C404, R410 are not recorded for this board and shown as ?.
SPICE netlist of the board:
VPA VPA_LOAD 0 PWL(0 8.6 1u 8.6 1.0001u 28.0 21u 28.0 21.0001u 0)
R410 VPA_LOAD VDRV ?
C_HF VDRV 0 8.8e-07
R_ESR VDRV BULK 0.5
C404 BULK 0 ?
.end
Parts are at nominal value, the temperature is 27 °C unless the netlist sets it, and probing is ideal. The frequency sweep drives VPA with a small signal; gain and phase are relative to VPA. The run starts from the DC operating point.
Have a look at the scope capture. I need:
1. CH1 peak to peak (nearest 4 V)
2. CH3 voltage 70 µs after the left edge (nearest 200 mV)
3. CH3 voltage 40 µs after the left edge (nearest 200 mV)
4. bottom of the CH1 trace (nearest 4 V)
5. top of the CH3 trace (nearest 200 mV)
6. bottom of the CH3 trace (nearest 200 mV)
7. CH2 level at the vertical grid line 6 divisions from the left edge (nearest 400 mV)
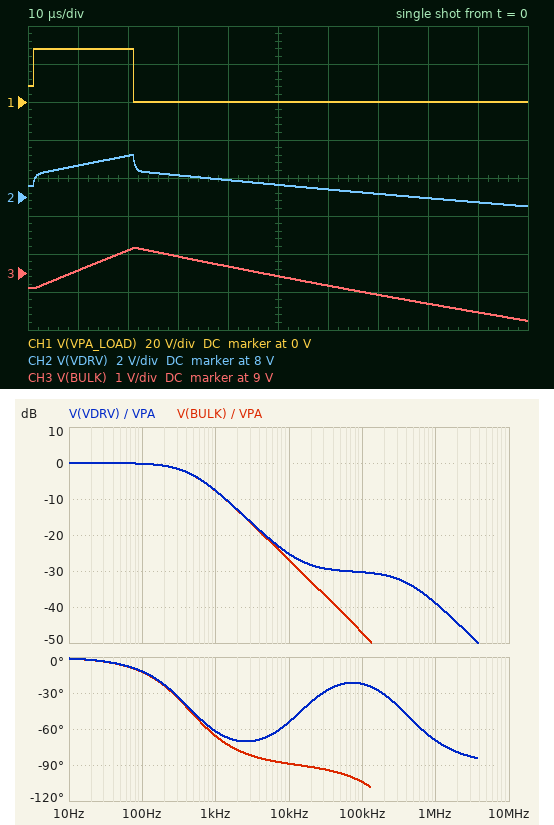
28 V
8.4 V
9.2 V
0 V
9.6 V
7.8 V
8.4 V
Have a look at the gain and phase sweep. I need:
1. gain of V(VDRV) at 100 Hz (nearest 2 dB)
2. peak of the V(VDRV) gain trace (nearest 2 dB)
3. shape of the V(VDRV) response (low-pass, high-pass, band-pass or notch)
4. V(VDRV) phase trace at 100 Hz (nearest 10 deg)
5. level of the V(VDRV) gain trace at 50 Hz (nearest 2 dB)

0 dB
0 dB
low-pass
-10 deg
0 dB
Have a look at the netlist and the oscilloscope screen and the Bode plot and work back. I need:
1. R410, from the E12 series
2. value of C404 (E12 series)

15 Ω
22 µF
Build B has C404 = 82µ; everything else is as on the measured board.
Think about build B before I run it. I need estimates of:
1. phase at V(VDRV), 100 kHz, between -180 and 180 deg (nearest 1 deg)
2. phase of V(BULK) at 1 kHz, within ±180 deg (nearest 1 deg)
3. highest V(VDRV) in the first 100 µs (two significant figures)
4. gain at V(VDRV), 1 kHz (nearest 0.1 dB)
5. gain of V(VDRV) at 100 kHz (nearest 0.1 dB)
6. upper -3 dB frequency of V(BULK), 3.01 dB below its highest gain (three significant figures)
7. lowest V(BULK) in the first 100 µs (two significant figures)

-17 deg
-83 deg
9.5 V
-17.9 dB
-30.2 dB
124 Hz
8.4 V
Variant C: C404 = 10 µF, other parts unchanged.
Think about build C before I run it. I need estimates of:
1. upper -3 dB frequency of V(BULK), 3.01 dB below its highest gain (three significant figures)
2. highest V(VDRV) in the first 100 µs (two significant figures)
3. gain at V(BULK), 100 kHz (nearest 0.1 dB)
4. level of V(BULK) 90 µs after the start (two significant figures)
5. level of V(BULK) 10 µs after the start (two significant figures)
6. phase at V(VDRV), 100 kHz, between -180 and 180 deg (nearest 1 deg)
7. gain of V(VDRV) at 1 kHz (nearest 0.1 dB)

948 Hz
11 V
-40.7 dB
7.2 V
9.6 V
-31 deg
-3.2 dB
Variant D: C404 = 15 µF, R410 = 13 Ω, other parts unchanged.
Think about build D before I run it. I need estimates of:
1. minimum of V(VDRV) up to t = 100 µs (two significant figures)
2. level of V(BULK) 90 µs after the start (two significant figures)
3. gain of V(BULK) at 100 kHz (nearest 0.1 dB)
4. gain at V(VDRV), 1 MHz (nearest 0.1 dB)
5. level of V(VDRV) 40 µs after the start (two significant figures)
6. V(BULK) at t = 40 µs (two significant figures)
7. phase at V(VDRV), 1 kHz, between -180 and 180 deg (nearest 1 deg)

6.9 V
7.5 V
-42.8 dB
-37.8 dB
9.1 V
9.5 V
-51 deg
